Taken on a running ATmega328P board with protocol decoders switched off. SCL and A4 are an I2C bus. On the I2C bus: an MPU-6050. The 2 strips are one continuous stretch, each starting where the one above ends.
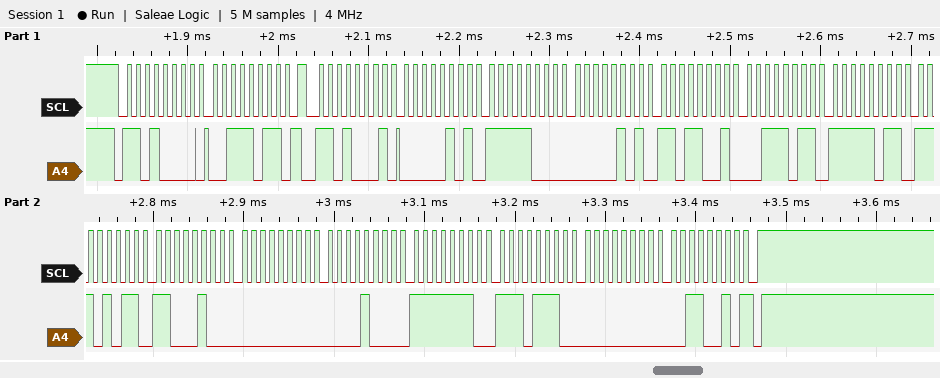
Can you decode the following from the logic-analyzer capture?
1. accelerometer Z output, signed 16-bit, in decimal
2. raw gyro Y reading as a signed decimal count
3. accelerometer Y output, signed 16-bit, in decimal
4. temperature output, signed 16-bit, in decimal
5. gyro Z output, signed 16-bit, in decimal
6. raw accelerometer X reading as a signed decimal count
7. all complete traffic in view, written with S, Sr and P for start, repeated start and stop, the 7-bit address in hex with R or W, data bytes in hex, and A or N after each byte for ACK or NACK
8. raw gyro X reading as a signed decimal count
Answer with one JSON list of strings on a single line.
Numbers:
["15355", "-274", "1497", "-5180", "50", "1528", "S 68W A 3B A Sr 68R A 05 A F8 A 05 A D9 A 3B A FB A EB A C4 A 00 A 08 A FE A EE A 00 A 32 N P", "8"]
